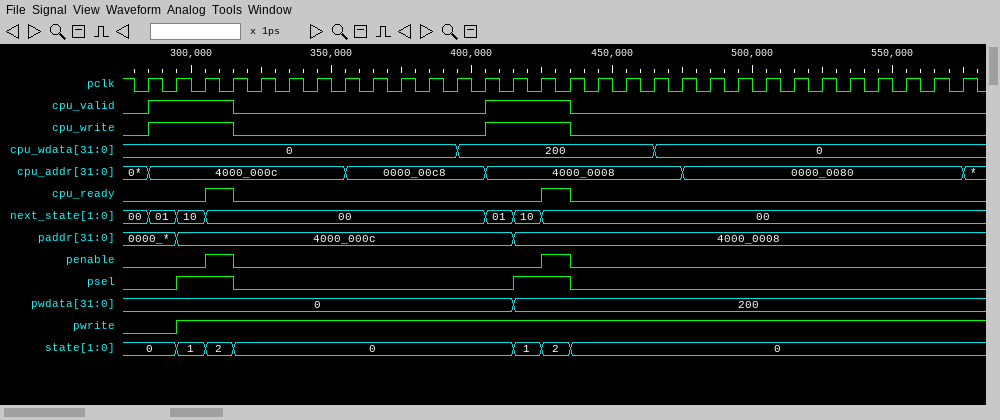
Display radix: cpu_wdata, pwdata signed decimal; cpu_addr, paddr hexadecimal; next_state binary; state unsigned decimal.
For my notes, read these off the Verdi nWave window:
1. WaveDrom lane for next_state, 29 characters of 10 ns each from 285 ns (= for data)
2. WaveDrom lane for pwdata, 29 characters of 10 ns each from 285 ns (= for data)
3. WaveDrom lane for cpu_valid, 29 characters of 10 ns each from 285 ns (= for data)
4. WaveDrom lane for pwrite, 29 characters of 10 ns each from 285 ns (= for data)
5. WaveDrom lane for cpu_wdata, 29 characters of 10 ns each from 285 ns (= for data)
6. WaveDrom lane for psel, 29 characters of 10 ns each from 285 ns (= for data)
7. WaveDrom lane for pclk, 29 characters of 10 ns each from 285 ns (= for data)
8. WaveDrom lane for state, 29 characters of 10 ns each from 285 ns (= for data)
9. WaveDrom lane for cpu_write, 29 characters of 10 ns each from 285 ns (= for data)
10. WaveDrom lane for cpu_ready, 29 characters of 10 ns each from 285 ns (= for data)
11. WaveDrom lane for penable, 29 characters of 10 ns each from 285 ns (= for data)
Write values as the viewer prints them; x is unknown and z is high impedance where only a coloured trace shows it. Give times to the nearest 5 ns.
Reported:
{name: 'next_state', wave: '===.........===..............', data: '01 10 00 01 10 00'}
{name: 'pwdata', wave: '=............=...............', data: '0 200'}
{name: 'cpu_valid', wave: '1..0........1..0.............'}
{name: 'pwrite', wave: '01...........................'}
{name: 'cpu_wdata', wave: '=..........=......=..........', data: '0 200 0'}
{name: 'psel', wave: '01.0.........1.0.............'}
{name: 'pclk', wave: 'p............................'}
{name: 'state', wave: '====.........===.............', data: '0 1 2 0 1 2 0'}
{name: 'cpu_write', wave: '1..0........1..0.............'}
{name: 'cpu_ready', wave: '0.10..........10.............'}
{name: 'penable', wave: '0.10..........10.............'}
